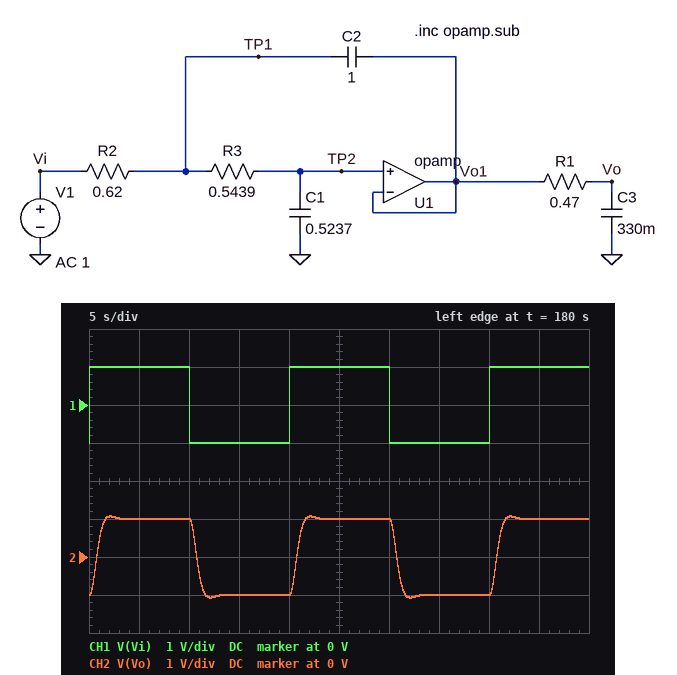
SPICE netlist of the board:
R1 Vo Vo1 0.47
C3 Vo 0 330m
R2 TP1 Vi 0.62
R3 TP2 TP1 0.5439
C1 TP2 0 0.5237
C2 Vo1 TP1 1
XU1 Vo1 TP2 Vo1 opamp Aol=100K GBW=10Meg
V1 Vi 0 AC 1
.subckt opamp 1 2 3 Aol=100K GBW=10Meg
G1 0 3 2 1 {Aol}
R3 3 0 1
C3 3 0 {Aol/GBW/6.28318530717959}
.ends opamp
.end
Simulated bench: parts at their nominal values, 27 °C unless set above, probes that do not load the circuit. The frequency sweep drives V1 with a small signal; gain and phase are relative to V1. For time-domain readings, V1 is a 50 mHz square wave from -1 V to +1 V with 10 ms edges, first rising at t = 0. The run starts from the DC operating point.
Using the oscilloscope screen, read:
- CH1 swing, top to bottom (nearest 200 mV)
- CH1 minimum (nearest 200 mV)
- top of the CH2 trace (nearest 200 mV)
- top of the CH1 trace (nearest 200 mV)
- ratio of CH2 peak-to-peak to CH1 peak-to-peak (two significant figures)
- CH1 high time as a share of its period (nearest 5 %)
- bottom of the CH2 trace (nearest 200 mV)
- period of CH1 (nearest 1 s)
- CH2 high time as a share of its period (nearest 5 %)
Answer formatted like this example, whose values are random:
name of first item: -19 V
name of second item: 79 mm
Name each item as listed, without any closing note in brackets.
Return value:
CH1 swing, top to bottom: 2.0 V
CH1 minimum: -1.0 V
top of the CH2 trace: 1.0 V
top of the CH1 trace: 1.0 V
ratio of CH2 peak-to-peak to CH1 peak-to-peak: 1.1
CH1 high time as a share of its period: 50 %
bottom of the CH2 trace: -1.0 V
period of CH1: 20 s
CH2 high time as a share of its period: 50 %
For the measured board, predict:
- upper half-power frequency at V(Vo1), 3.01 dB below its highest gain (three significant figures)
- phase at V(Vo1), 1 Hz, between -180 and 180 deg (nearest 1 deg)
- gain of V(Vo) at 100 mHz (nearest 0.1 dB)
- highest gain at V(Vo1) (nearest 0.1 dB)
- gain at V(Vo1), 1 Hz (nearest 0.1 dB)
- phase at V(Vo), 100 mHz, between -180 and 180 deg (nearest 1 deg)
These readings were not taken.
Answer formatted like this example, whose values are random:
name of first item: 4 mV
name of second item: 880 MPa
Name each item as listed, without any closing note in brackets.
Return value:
upper half-power frequency at V(Vo1), 3.01 dB below its highest gain: 369 mHz
phase at V(Vo1), 1 Hz, between -180 and 180 deg: -147 deg
gain of V(Vo) at 100 mHz: -0.1 dB
highest gain at V(Vo1): 0 dB
gain at V(Vo1), 1 Hz: -17.0 dB
phase at V(Vo), 100 mHz, between -180 and 180 deg: -28 deg
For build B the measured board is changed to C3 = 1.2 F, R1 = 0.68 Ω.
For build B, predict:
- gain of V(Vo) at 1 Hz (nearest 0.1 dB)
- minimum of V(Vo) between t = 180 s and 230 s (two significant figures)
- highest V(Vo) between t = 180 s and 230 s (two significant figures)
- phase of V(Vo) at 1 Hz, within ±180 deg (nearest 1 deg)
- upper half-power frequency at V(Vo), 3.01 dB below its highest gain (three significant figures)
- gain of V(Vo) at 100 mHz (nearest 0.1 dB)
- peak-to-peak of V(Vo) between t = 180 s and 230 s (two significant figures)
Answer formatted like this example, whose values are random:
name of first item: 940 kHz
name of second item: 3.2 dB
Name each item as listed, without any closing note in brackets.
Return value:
gain of V(Vo) at 1 Hz: -31.4 dB
minimum of V(Vo) between t = 180 s and 230 s: -1.0 V
highest V(Vo) between t = 180 s and 230 s: 1.0 V
phase of V(Vo) at 1 Hz, within ±180 deg: 134 deg
upper half-power frequency at V(Vo), 3.01 dB below its highest gain: 181 mHz
gain of V(Vo) at 100 mHz: -1.1 dB
peak-to-peak of V(Vo) between t = 180 s and 230 s: 2.0 V
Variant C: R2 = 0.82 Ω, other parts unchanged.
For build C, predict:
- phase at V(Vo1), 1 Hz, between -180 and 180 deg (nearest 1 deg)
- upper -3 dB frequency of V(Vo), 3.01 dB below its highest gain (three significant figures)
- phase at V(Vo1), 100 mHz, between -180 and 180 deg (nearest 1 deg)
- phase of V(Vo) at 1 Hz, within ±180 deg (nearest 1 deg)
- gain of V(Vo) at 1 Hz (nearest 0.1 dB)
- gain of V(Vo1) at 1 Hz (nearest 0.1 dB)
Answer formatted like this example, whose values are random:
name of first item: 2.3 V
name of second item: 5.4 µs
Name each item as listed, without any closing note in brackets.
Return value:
phase at V(Vo1), 1 Hz, between -180 and 180 deg: -151 deg
upper -3 dB frequency of V(Vo), 3.01 dB below its highest gain: 300 mHz
phase at V(Vo1), 100 mHz, between -180 and 180 deg: -26 deg
phase of V(Vo) at 1 Hz, within ±180 deg: 164 deg
gain of V(Vo) at 1 Hz: -22.3 dB
gain of V(Vo1) at 1 Hz: -19.4 dB
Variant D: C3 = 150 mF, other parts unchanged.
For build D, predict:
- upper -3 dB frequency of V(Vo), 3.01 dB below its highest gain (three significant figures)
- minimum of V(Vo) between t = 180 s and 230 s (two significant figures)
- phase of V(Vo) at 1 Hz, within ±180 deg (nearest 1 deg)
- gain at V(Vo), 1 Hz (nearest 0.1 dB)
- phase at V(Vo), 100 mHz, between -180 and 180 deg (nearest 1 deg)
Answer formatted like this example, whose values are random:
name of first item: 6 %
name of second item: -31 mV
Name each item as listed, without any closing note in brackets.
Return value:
upper -3 dB frequency of V(Vo), 3.01 dB below its highest gain: 364 mHz
minimum of V(Vo) between t = 180 s and 230 s: -1.1 V
phase of V(Vo) at 1 Hz, within ±180 deg: -171 deg
gain at V(Vo), 1 Hz: -17.8 dB
phase at V(Vo), 100 mHz, between -180 and 180 deg: -25 deg
